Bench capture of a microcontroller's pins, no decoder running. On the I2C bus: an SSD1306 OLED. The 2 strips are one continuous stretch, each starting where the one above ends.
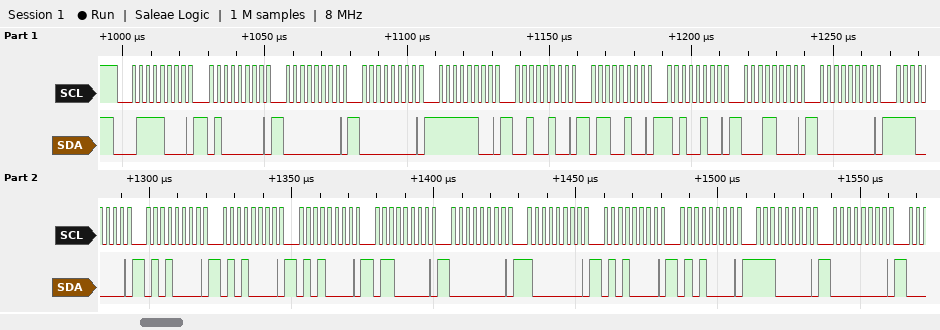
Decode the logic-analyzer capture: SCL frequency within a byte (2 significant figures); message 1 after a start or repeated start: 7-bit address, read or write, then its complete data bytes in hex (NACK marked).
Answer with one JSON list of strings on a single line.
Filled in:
["400 kHz", "0x3C write: 40 00 00 FC 24 64 A4 18 00 E0 50 50 50 60 00 80 50 50 E0 00"]
